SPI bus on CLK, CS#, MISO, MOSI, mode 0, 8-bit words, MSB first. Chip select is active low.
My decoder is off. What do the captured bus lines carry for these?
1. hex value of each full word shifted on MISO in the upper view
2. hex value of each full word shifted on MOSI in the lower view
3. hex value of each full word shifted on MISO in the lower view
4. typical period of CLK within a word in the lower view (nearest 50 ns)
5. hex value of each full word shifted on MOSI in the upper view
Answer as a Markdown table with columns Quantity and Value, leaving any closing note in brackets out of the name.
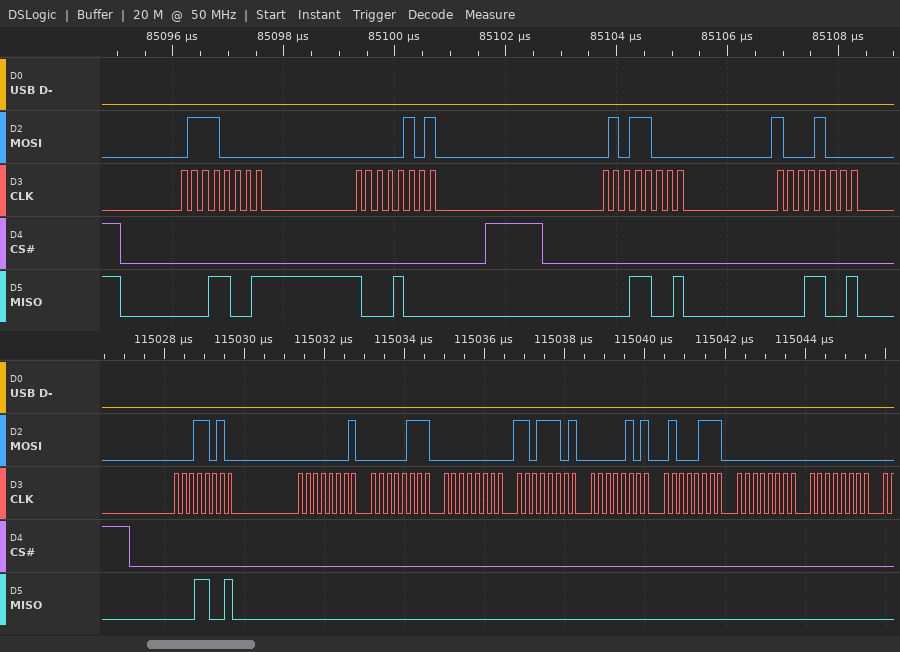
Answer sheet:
| Quantity | Value |
|---|---|
| hex value of each full word shifted on MISO in the upper view | 19, 88, 19, 19 |
| hex value of each full word shifted on MOSI in the lower view | 1A, 01, 07, 00, DD, 05, 47, 00, 00 |
| hex value of each full word shifted on MISO in the lower view | 19, 00, 00, 00, 00, 00, 00, 00, 00 |
| typical period of CLK within a word in the lower view | 200 ns |
| hex value of each full word shifted on MOSI in the upper view | 70, 05, 58, 88 |
